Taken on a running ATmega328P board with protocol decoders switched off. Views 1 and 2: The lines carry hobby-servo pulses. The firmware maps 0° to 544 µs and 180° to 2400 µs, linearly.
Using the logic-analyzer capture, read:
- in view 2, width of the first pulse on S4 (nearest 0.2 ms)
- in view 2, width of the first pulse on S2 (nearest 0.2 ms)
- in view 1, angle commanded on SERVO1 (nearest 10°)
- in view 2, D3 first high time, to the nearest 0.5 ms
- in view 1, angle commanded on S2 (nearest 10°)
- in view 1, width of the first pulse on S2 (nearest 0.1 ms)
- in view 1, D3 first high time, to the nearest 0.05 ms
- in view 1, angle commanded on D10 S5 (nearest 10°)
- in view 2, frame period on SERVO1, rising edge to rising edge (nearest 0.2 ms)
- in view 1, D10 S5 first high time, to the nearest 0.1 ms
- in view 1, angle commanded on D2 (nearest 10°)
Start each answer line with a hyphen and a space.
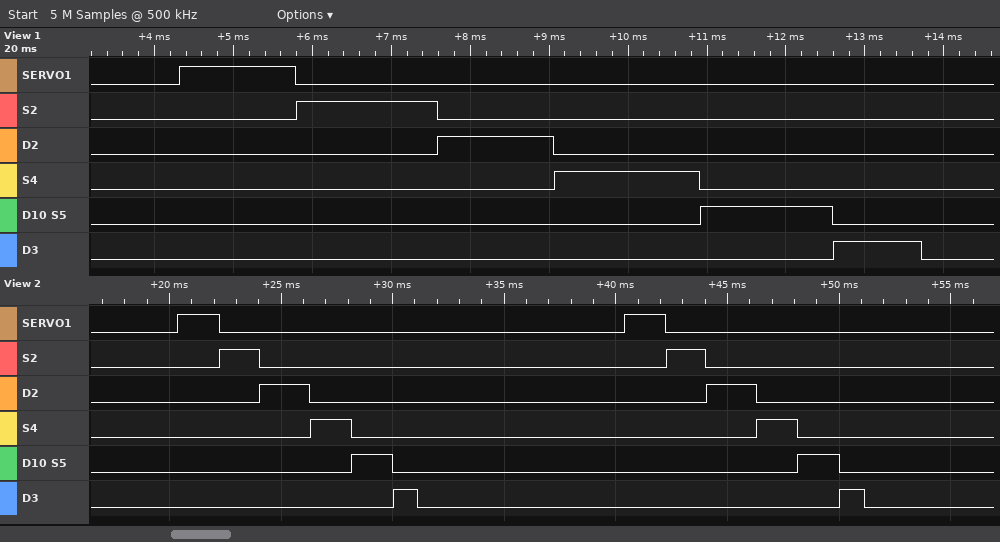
- 1.8 ms
- 1.8 ms
- 90°
- 1.0 ms
- 120°
- 1.8 ms
- 1.10 ms
- 110°
- 20.0 ms
- 1.7 ms
- 90°
